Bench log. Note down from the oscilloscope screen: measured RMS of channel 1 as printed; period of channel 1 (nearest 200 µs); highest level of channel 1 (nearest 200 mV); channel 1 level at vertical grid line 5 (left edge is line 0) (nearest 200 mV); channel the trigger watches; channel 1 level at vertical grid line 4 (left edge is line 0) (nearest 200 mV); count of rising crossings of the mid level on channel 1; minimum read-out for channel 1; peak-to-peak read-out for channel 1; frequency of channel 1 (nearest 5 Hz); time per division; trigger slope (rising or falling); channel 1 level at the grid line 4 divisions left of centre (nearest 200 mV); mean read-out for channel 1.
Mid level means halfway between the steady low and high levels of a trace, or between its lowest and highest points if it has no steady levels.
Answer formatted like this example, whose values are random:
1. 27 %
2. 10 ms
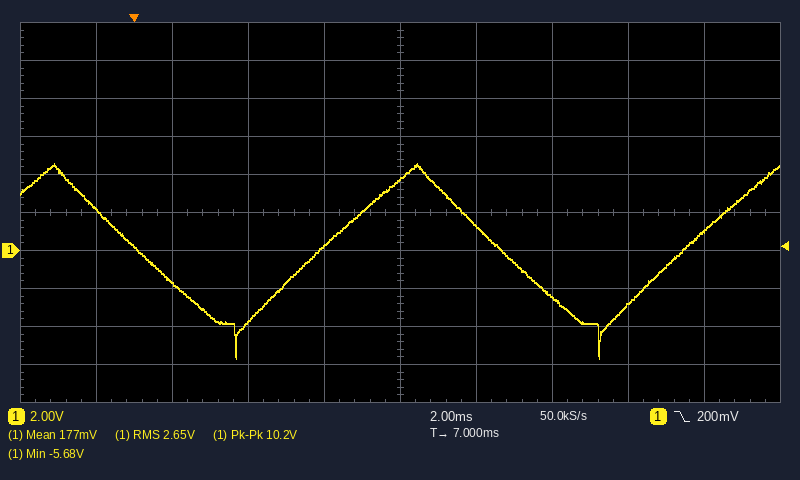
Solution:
1. 2.65 V
2. 9.6 ms
3. 4.6 V
4. 3.8 V
5. channel 1
6. 200 mV
7. 2
8. -5.68 V
9. 10.2 V
10. 105 Hz
11. 2 ms
12. falling
13. 2.2 V
14. 177 mV
